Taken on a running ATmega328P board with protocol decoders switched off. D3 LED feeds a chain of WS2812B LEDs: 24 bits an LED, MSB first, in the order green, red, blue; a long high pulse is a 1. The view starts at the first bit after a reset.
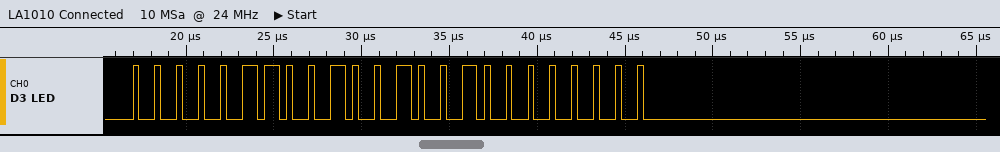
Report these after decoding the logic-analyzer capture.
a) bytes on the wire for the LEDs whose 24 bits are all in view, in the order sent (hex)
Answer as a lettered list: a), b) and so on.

a) 06 49 00
